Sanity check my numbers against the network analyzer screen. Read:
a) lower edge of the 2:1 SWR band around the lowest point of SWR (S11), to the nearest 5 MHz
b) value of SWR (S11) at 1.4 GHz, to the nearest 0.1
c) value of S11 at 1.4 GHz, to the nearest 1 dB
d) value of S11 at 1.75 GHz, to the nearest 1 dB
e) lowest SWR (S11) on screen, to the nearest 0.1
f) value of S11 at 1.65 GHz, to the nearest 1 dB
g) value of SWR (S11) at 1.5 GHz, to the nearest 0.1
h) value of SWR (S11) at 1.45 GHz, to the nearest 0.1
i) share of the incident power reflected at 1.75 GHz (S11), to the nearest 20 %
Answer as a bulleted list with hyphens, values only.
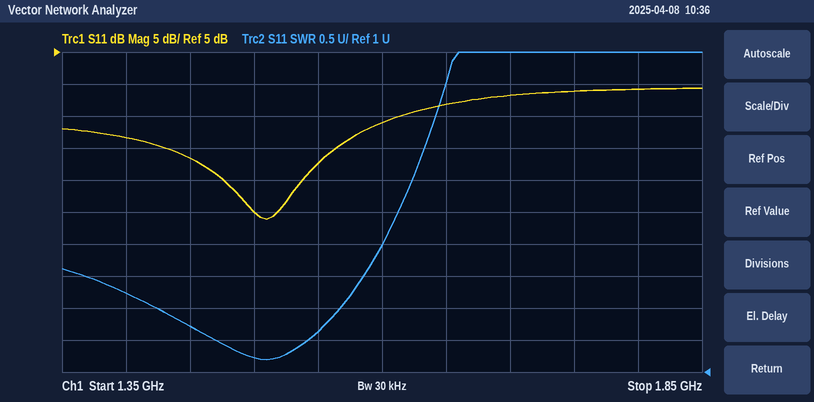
- 1.425 GHz
- 2.2
- -8 dB
- -1 dB
- 1.2
- -3 dB
- 1.2
- 1.7
- 80 %
